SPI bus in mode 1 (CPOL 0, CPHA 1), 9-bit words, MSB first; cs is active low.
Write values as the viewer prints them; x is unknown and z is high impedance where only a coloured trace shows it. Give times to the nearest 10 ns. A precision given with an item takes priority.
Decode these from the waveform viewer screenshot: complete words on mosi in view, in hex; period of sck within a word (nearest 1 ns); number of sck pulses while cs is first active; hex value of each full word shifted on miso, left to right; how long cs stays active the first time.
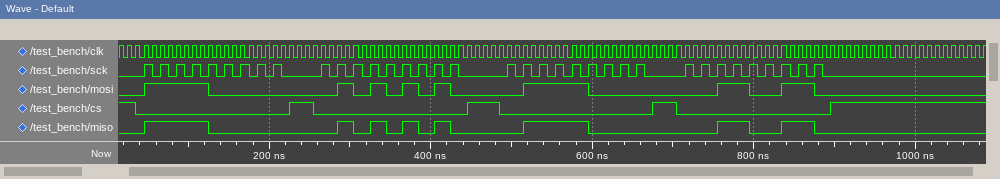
1E0, 0AA, 0F0, 066
20 ns
9
1E0, 0AA, 0F0, 066
190 ns
